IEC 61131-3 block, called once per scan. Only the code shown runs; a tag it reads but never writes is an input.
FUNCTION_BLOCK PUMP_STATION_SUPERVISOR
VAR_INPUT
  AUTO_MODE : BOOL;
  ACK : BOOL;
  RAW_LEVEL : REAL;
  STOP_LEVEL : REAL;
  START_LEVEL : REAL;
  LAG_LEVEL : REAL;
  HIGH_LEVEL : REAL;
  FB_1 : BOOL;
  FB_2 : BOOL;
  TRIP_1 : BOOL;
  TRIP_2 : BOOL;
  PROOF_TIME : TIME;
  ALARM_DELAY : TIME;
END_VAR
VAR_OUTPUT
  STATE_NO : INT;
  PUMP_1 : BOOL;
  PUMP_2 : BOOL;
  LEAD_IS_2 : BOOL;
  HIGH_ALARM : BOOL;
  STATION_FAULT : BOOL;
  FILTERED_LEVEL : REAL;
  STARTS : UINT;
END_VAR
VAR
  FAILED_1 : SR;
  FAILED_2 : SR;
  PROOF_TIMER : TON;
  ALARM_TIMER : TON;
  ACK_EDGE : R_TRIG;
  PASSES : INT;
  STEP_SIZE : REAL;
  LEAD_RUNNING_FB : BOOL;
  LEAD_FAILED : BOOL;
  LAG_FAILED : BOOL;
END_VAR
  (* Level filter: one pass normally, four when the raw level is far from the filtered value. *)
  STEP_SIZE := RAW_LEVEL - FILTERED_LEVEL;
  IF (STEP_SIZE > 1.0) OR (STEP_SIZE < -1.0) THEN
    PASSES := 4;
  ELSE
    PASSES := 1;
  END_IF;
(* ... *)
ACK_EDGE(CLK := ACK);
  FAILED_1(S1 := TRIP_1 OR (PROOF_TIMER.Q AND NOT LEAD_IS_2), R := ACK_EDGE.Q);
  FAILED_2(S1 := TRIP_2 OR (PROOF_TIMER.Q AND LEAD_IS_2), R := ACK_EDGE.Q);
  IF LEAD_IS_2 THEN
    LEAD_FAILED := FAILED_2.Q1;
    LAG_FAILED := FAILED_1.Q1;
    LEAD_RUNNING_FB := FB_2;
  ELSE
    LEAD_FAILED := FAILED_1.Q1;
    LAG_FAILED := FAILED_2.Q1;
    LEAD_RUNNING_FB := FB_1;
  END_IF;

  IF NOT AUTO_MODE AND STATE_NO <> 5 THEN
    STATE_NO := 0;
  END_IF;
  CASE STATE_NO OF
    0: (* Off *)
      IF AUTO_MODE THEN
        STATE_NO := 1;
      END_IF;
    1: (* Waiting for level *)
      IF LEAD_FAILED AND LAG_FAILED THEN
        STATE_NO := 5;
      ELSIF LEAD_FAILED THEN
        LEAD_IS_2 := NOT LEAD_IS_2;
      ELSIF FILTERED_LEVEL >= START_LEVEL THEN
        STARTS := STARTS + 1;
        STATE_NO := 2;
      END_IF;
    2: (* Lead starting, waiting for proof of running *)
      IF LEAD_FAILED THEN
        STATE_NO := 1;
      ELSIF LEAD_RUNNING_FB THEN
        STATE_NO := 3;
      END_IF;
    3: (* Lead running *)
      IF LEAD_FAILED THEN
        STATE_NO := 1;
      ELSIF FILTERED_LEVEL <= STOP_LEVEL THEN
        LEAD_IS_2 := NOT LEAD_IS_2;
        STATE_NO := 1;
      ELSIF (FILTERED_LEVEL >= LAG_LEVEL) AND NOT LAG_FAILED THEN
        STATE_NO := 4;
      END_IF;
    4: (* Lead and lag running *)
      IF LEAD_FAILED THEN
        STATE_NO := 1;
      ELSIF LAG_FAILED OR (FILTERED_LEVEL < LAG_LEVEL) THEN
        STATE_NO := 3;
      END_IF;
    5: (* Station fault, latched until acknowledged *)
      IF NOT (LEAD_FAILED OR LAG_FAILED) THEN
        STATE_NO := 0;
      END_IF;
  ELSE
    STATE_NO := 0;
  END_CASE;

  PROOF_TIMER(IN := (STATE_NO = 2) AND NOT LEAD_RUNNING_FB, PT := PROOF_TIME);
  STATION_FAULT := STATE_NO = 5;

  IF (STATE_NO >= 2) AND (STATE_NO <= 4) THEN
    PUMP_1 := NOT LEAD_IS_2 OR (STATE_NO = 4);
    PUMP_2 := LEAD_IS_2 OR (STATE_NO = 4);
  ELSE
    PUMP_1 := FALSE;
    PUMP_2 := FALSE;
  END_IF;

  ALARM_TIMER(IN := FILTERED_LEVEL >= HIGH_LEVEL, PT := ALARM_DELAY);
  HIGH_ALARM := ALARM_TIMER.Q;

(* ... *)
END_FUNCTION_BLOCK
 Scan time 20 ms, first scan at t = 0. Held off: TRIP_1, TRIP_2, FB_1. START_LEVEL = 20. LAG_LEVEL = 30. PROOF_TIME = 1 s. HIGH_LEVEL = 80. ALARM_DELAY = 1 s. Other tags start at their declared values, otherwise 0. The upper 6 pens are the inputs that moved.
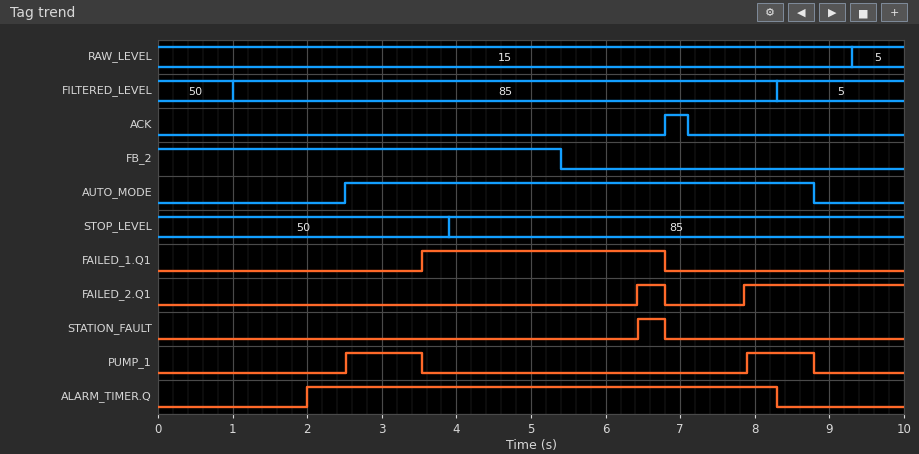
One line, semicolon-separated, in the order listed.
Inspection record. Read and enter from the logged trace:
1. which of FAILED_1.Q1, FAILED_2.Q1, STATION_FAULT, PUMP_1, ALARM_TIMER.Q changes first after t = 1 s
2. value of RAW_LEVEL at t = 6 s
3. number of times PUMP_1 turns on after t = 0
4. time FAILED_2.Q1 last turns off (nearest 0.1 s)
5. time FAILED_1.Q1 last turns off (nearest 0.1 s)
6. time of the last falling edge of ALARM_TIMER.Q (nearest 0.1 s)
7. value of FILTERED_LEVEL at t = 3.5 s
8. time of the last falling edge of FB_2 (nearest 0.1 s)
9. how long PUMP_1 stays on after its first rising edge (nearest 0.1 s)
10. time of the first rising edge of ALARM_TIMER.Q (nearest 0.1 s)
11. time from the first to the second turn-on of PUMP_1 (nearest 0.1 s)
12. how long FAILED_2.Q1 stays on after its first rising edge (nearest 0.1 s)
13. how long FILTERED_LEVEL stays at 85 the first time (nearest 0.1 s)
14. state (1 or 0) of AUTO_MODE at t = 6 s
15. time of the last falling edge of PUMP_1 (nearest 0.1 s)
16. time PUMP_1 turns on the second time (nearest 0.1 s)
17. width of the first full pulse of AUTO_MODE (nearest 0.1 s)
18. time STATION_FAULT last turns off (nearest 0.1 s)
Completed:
ALARM_TIMER.Q; 15; 2; 6.8 s; 6.8 s; 8.3 s; 85; 5.4 s; 1.0 s; 2.0 s; 5.4 s; 0.4 s; 7.3 s; 1; 8.8 s; 7.9 s; 6.3 s; 6.8 s
